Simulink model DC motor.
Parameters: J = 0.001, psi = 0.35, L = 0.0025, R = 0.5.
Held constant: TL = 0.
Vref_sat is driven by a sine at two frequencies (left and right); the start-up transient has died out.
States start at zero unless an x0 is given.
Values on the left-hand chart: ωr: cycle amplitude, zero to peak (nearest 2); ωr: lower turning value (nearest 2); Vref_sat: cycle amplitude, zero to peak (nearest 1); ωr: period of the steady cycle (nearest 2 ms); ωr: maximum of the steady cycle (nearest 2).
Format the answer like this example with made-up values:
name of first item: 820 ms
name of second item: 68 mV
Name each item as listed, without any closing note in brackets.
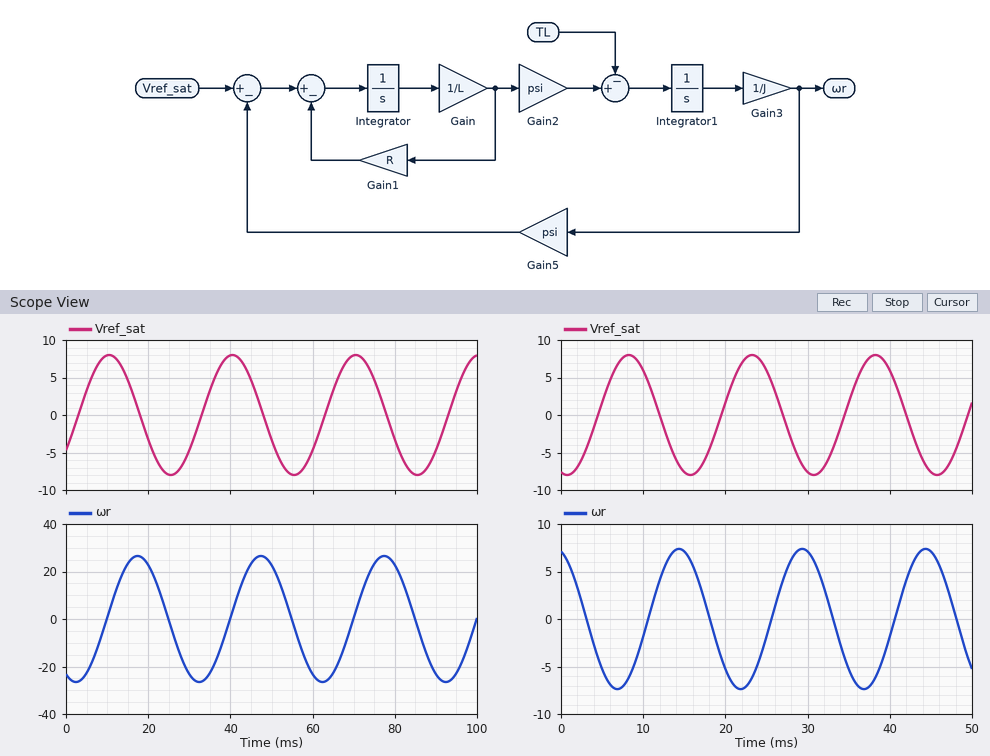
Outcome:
ωr: cycle amplitude, zero to peak: 26
ωr: lower turning value: -26
Vref_sat: cycle amplitude, zero to peak: 8
ωr: period of the steady cycle: 30 ms
ωr: maximum of the steady cycle: 26
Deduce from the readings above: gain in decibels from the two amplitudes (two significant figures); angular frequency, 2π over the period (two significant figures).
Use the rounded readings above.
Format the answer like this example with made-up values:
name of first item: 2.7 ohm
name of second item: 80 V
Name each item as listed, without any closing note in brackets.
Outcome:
gain in decibels from the two amplitudes: 10 dB
angular frequency, 2π over the period: 0.21 rad/ms
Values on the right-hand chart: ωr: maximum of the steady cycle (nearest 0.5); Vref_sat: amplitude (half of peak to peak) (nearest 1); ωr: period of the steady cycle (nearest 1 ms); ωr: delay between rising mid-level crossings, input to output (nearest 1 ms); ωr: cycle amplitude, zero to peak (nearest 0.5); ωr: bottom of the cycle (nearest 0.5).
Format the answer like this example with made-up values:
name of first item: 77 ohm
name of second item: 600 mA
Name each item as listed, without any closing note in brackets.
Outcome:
ωr: maximum of the steady cycle: 7.5
Vref_sat: amplitude (half of peak to peak): 8
ωr: period of the steady cycle: 15 ms
ωr: delay between rising mid-level crossings, input to output: 6 ms
ωr: cycle amplitude, zero to peak: 7.5
ωr: bottom of the cycle: -7.5
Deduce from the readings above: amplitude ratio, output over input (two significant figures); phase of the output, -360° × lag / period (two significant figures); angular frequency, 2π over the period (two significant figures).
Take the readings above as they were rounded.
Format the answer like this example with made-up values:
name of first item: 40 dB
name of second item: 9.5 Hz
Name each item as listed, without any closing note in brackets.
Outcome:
amplitude ratio, output over input: 0.94
phase of the output, -360° × lag / period: -140°
angular frequency, 2π over the period: 0.42 rad/ms
